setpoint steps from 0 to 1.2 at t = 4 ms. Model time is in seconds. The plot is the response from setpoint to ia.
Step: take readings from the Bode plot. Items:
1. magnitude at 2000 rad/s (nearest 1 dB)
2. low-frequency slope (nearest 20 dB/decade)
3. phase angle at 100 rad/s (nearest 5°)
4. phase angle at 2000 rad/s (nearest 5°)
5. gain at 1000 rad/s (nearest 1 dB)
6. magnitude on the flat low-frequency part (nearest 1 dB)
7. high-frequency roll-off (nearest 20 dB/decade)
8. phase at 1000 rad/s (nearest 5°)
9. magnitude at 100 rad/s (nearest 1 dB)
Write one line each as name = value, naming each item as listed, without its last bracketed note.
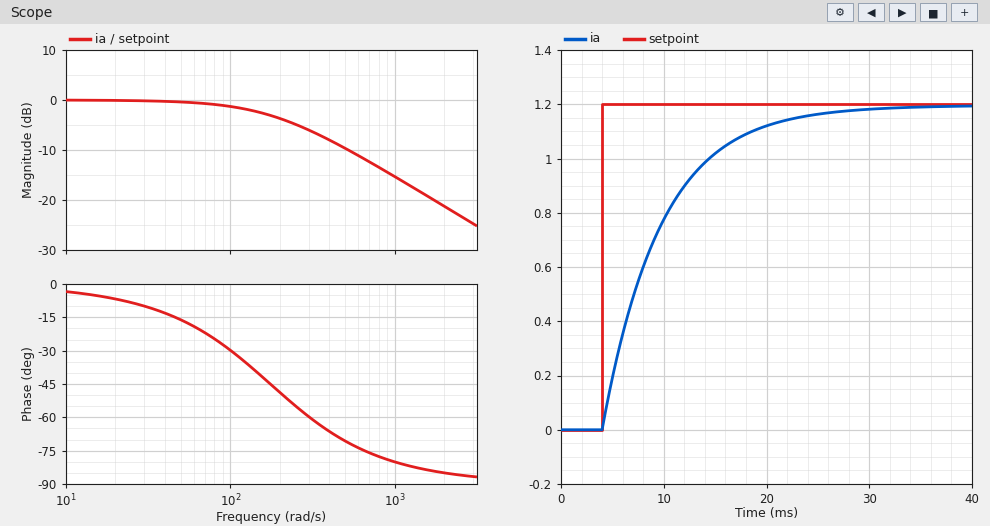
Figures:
magnitude at 2000 rad/s = -21 dB
low-frequency slope = 0 dB/decade
phase angle at 100 rad/s = -30°
phase angle at 2000 rad/s = -85°
gain at 1000 rad/s = -15 dB
magnitude on the flat low-frequency part = 0 dB
high-frequency roll-off = -20 dB/decade
phase at 1000 rad/s = -80°
magnitude at 100 rad/s = -1 dB
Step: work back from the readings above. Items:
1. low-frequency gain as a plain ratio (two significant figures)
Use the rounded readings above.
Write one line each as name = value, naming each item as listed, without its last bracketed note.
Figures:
low-frequency gain as a plain ratio = 1.0
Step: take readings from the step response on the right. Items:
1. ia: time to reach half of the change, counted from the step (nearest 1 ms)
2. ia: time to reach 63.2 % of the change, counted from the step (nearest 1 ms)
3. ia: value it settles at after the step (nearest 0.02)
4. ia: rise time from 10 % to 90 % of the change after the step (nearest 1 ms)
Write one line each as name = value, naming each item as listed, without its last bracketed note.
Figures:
ia: time to reach half of the change, counted from the step = 4 ms
ia: time to reach 63.2 % of the change, counted from the step = 6 ms
ia: value it settles at after the step = 1.20
ia: rise time from 10 % to 90 % of the change after the step = 13 ms
